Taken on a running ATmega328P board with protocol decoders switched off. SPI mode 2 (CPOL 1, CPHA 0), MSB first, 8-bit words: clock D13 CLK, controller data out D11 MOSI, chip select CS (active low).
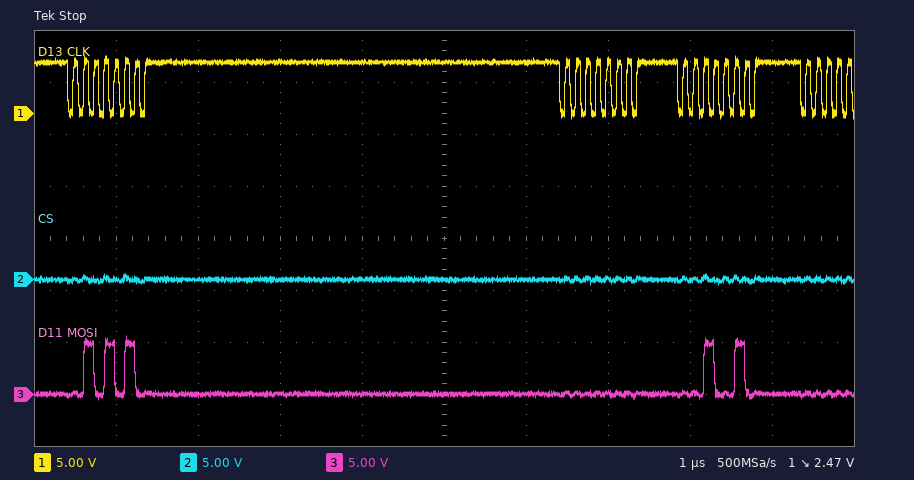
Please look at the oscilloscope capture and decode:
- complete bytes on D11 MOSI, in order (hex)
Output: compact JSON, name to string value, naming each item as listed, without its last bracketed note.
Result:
{"complete bytes on D11 MOSI, in order": "2A 00 12"}
